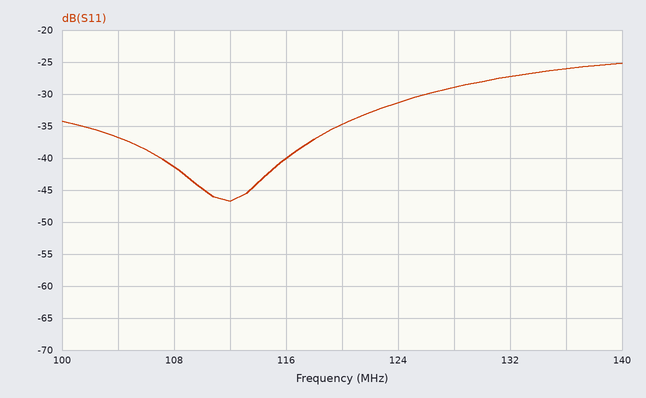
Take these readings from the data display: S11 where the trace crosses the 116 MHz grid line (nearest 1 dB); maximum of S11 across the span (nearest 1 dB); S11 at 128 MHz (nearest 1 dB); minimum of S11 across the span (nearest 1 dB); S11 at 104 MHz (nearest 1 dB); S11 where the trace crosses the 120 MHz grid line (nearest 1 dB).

-40 dB
-25 dB
-29 dB
-47 dB
-37 dB
-35 dB
